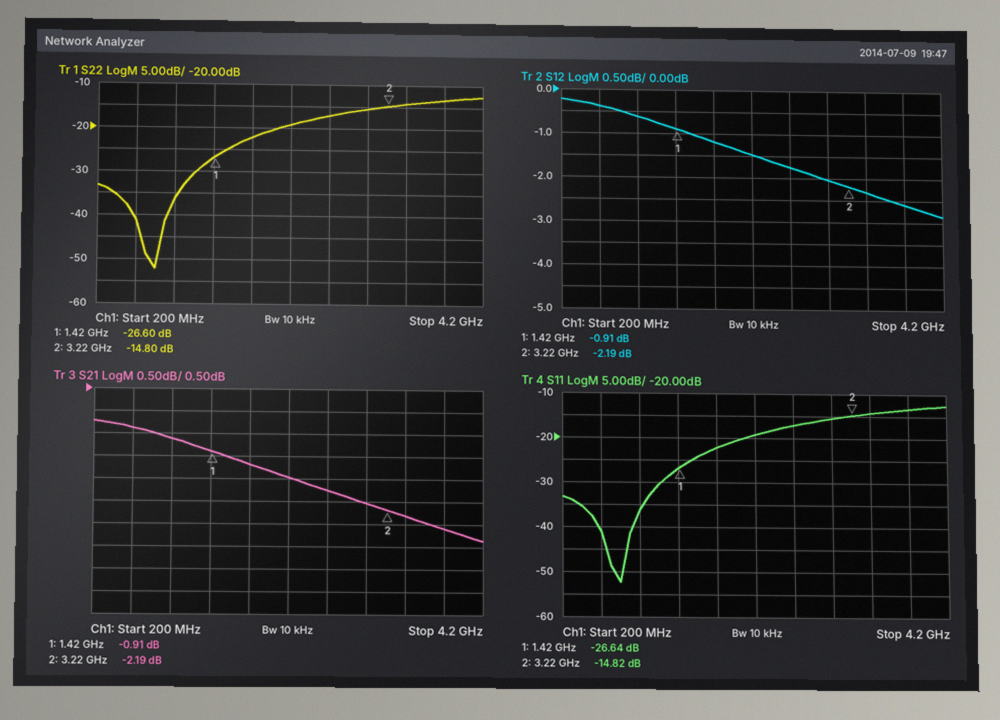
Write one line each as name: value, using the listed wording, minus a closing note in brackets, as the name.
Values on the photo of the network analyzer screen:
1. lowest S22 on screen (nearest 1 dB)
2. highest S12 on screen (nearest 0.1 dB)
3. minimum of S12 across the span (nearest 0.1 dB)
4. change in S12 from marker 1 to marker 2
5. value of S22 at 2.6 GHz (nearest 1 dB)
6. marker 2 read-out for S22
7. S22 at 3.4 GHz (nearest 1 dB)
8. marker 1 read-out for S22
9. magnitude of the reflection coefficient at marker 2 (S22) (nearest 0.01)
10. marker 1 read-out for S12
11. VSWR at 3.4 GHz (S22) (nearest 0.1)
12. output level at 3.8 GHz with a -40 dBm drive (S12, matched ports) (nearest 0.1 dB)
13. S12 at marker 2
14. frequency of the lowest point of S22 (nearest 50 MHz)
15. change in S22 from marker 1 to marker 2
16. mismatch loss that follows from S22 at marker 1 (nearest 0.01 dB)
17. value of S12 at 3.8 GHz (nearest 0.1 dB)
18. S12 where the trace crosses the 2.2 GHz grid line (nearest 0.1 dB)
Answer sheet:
lowest S22 on screen: -52 dB
highest S12 on screen: -0.2 dB
minimum of S12 across the span: -2.9 dB
change in S12 from marker 1 to marker 2: -1.28 dB
value of S22 at 2.6 GHz: -17 dB
marker 2 read-out for S22: -14.80 dB
S22 at 3.4 GHz: -14 dB
marker 1 read-out for S22: -26.60 dB
magnitude of the reflection coefficient at marker 2 (S22): 0.18
marker 1 read-out for S12: -0.91 dB
VSWR at 3.4 GHz (S22): 1.5
output level at 3.8 GHz with a -40 dBm drive (S12, matched ports): -42.6 dBm
S12 at marker 2: -2.19 dB
frequency of the lowest point of S22: 800 MHz
change in S22 from marker 1 to marker 2: 11.80 dB
mismatch loss that follows from S22 at marker 1: 0.01 dB
value of S12 at 3.8 GHz: -2.6 dB
S12 where the trace crosses the 2.2 GHz grid line: -1.5 dB
